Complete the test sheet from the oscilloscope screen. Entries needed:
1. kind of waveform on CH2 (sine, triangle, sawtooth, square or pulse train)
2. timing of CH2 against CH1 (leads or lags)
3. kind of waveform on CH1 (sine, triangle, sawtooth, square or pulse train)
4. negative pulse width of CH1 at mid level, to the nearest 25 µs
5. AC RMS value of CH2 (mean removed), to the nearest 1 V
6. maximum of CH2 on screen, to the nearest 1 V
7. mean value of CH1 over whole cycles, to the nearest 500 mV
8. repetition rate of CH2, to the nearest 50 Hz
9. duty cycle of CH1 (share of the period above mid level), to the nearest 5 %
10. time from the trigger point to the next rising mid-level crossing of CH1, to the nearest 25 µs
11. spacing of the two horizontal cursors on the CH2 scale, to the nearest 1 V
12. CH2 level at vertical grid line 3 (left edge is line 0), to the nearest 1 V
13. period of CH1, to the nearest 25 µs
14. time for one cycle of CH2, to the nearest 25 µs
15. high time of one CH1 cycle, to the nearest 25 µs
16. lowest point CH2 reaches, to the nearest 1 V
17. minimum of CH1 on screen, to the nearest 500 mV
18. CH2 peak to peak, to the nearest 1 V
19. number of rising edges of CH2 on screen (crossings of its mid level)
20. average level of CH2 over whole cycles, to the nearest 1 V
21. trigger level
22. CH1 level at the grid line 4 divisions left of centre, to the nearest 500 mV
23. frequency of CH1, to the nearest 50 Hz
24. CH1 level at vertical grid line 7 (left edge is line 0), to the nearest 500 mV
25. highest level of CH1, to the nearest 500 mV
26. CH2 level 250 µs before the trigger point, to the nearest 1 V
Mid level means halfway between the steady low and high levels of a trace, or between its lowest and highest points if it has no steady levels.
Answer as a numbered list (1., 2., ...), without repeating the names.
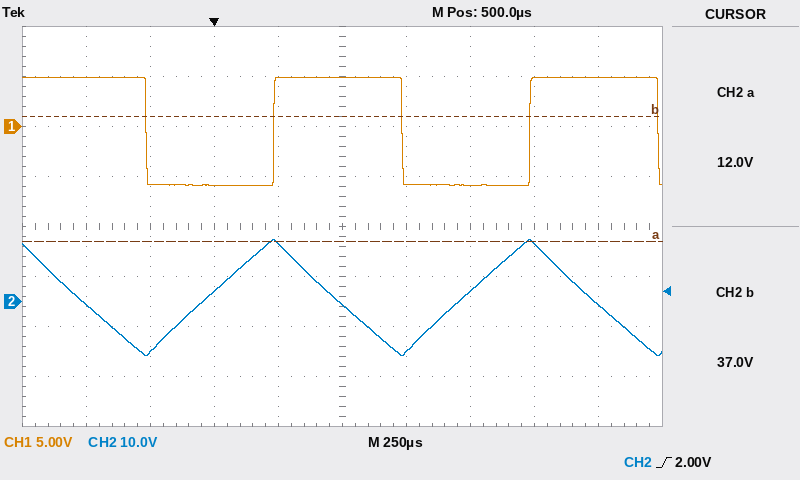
1. triangle
2. leads
3. square
4. 500 µs
5. 7 V
6. 12 V
7. -500 mV
8. 1.00 kHz
9. 50 %
10. 225 µs
11. 25 V
12. 2 V
13. 1.000 ms
14. 1.000 ms
15. 500 µs
16. -11 V
17. -6.0 V
18. 23 V
19. 2
20. 1 V
21. 2.00 V
22. 5.0 V
23. 1.00 kHz
24. -6.0 V
25. 5.0 V
26. -10 V
